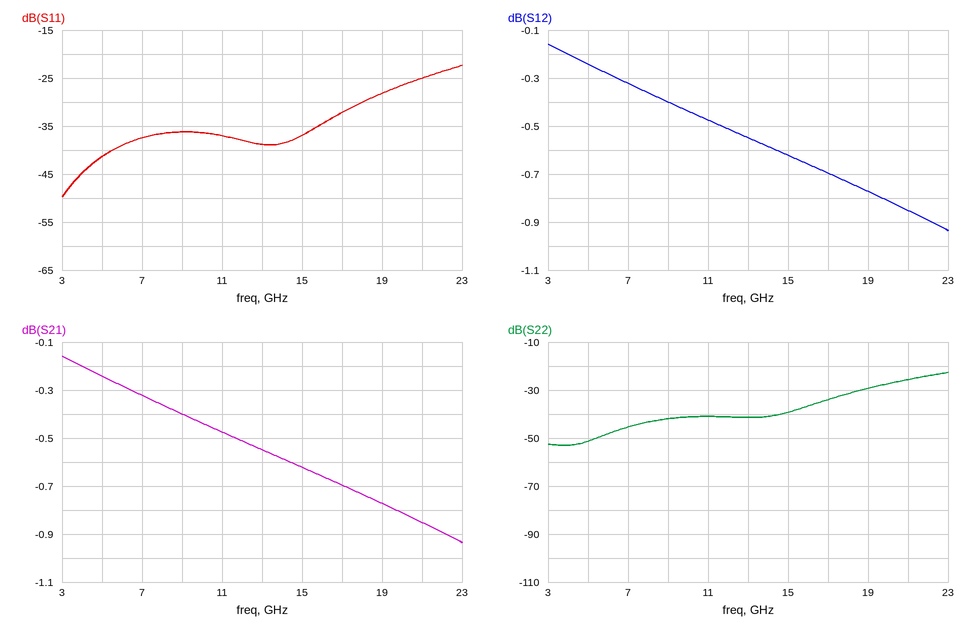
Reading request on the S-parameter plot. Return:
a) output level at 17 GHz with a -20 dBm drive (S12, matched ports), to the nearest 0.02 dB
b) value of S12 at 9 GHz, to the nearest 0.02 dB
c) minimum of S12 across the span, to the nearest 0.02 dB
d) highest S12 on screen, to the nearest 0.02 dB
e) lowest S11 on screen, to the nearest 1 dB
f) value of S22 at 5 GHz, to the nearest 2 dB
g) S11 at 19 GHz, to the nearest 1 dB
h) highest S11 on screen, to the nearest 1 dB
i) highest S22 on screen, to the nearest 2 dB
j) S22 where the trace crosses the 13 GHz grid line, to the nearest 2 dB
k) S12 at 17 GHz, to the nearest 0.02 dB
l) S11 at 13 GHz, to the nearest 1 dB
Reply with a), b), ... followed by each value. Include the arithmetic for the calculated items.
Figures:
a) -20 dBm + (-0.70 dB) = -20.70 dBm
b) -0.40 dB
c) -0.94 dB
d) -0.16 dB
e) -50 dB
f) -52 dB
g) -28 dB
h) -22 dB
i) -22 dB
j) -42 dB
k) -0.70 dB
l) -39 dB
